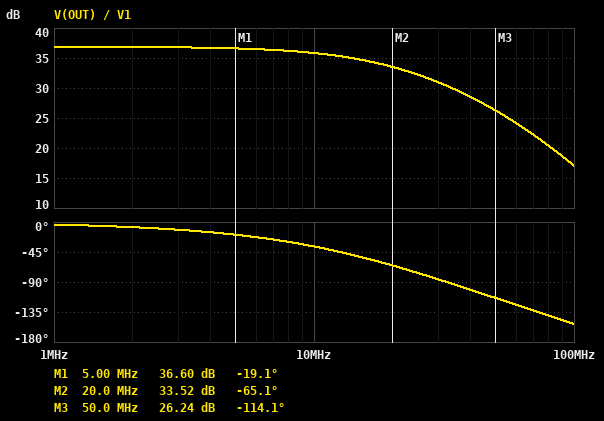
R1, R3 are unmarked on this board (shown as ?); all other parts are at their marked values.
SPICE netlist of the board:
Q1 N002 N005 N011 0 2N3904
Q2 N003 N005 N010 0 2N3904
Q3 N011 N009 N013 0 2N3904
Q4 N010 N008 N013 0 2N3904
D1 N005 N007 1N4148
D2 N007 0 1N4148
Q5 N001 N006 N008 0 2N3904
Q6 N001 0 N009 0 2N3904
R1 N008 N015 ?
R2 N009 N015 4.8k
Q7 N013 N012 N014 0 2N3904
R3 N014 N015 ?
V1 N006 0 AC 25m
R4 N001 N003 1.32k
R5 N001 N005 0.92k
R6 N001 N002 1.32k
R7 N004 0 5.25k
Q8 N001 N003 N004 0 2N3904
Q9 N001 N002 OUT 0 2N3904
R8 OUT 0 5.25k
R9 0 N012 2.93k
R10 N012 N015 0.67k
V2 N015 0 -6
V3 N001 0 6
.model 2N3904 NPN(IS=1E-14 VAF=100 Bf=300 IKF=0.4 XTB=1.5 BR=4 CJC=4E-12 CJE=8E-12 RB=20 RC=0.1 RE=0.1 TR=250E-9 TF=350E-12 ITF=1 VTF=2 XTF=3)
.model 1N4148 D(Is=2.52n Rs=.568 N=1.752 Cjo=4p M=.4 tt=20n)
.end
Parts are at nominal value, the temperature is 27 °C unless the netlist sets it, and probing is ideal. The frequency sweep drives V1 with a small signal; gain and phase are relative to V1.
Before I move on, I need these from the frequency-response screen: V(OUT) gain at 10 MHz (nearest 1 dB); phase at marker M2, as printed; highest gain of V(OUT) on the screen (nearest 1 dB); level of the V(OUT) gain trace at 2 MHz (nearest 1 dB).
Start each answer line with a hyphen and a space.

- 36 dB
- -65.1 deg
- 37 dB
- 37 dB
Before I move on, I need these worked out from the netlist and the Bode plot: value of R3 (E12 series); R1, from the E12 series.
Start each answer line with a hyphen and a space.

- 68 Ω
- 3.9 kΩ
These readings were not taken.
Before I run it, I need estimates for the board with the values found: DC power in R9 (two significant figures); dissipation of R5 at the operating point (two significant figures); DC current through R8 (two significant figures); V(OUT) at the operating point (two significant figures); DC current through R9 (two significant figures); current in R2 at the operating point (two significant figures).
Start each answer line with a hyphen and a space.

- 8.2 mW
- 24 mW
- 210 µA
- 1.1 V
- 1.7 mA
- 1.1 mA
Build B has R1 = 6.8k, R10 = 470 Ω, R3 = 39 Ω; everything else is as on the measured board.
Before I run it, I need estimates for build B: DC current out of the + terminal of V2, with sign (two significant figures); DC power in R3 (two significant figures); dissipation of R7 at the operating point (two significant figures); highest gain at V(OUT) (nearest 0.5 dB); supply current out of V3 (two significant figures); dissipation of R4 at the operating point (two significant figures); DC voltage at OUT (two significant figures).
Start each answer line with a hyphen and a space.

- -7.2 mA
- 480 µW
- 1.4 mW
- 32.5 dB
- 12 mA
- 5.5 mW
- 3.4 V
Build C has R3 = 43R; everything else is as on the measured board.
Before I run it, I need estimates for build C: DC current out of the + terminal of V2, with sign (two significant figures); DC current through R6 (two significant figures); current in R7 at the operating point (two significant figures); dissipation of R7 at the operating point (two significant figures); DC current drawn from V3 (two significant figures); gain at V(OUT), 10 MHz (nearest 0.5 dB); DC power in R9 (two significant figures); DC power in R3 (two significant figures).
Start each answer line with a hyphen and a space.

- -13 mA
- 4.1 mA
- 29 µA
- 4.4 µW
- 16 mA
- 2.5 dB
- 8.2 mW
- 3.5 mW
